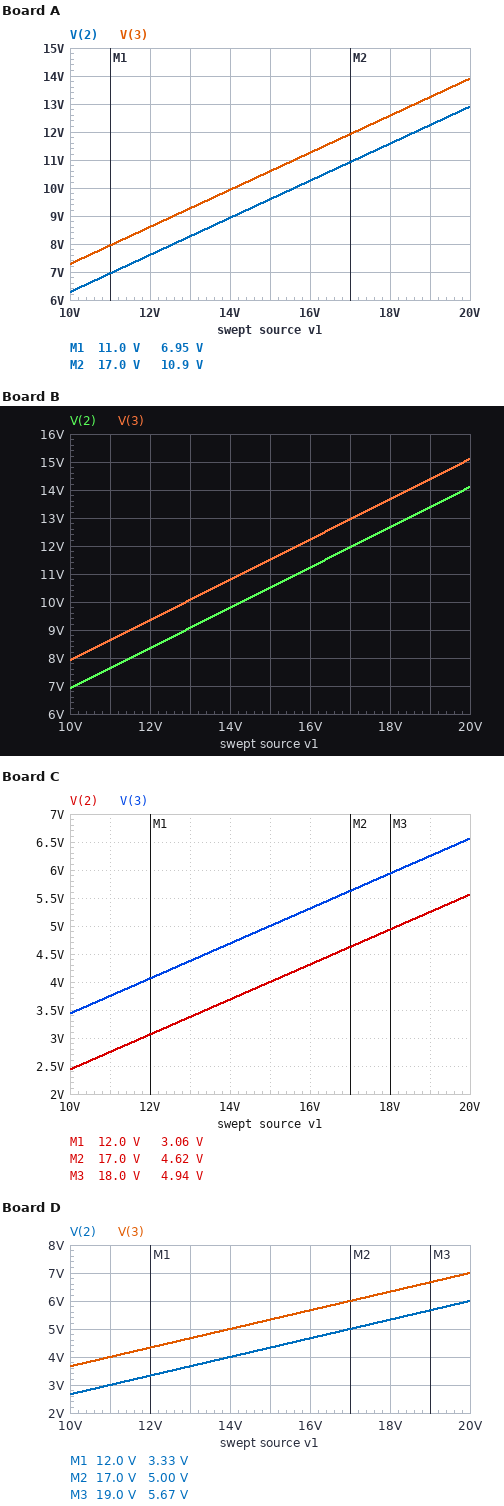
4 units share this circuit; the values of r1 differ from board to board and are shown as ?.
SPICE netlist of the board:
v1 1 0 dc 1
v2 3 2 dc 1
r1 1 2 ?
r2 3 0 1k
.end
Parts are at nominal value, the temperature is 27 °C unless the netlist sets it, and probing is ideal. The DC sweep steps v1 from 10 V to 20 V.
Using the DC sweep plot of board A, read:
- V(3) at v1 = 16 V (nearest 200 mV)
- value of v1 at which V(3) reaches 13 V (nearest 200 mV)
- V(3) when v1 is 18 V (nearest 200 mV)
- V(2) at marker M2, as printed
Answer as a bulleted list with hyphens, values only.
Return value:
- 11.2 V
- 18.6 V
- 12.6 V
- 10.9 V
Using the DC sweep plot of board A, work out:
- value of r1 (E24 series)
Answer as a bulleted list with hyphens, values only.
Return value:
- 510 Ω
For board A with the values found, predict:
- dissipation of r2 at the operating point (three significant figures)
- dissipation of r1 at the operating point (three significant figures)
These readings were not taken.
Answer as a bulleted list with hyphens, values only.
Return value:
- 1.75 mW
- 895 µW
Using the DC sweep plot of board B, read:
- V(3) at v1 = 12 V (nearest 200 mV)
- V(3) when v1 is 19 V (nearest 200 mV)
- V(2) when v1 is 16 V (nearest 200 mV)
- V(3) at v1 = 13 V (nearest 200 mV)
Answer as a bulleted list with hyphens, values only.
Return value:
- 9.4 V
- 14.4 V
- 11.2 V
- 10.0 V
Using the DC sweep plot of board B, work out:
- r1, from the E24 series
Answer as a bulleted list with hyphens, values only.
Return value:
- 390 Ω
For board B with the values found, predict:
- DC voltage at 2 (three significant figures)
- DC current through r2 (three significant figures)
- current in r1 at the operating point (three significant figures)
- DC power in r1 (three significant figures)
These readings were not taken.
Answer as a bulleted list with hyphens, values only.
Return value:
- 439 mV
- 1.44 mA
- 1.44 mA
- 807 µW
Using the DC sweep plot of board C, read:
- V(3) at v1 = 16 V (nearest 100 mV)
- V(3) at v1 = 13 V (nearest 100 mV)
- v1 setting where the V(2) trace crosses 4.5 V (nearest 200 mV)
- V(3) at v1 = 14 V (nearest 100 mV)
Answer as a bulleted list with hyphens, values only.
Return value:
- 5.3 V
- 4.4 V
- 16.6 V
- 4.7 V
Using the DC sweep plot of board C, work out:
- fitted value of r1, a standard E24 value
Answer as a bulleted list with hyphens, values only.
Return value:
- 2.2 kΩ
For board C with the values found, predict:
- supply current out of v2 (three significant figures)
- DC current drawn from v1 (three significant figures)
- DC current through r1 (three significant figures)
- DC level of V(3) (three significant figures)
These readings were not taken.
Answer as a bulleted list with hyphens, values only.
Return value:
- 625 µA
- 625 µA
- 625 µA
- 625 mV
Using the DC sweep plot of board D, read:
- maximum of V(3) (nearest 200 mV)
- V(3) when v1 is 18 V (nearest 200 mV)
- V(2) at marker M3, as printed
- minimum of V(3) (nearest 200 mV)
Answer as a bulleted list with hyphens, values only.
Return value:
- 7.0 V
- 6.4 V
- 5.67 V
- 3.6 V
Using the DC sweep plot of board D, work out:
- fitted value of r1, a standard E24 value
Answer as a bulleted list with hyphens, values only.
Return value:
- 2 kΩ
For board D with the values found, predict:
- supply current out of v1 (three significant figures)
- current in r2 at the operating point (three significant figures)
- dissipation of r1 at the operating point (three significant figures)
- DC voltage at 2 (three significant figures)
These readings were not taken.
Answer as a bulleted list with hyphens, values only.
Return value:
- 667 µA
- 667 µA
- 889 µW
- -333 mV
